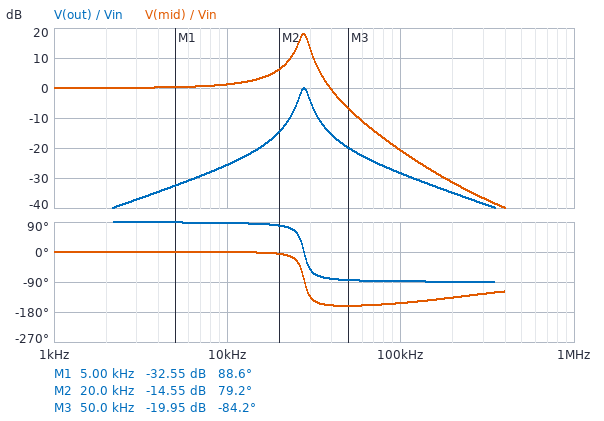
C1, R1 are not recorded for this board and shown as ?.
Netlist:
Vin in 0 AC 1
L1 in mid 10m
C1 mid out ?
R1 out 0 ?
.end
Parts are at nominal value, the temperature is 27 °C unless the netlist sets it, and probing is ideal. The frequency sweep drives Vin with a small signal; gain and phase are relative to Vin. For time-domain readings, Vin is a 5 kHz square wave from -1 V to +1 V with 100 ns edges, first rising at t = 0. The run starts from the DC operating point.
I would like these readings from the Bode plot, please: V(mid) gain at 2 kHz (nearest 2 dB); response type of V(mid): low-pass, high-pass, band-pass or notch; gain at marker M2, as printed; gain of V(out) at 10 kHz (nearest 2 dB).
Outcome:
0 dB
low-pass
-14.55 dB
-26 dB
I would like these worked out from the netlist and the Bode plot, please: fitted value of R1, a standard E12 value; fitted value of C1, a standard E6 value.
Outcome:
220 Ω
3.3 nF
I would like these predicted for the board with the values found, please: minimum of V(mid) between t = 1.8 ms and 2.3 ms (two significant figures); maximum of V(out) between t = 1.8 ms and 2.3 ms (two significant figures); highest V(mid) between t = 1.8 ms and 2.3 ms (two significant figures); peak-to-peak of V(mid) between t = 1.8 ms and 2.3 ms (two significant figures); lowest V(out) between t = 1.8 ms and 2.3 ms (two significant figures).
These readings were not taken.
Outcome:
-2.6 V
220 mV
2.6 V
5.1 V
-220 mV
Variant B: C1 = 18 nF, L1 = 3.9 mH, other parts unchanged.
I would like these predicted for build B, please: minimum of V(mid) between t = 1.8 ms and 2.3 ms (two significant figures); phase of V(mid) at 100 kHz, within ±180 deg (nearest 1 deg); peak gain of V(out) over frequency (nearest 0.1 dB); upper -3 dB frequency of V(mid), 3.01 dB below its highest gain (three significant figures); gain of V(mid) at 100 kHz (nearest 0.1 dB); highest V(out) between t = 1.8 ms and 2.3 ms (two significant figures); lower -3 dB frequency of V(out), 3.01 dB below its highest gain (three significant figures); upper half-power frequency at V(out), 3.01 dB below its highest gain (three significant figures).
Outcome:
-2.0 V
-107 deg
0 dB
22.4 kHz
-20.0 dB
670 mV
15.0 kHz
24.0 kHz
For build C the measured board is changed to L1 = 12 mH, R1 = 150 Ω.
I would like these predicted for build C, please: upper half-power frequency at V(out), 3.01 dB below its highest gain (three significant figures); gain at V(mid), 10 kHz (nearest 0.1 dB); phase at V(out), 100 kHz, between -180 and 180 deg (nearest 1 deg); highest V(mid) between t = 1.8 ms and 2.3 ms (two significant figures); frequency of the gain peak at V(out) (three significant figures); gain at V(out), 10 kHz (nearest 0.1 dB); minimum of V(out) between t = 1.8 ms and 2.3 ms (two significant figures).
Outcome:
26.3 kHz
1.5 dB
-89 deg
4.7 V
25.3 kHz
-28.7 dB
-310 mV
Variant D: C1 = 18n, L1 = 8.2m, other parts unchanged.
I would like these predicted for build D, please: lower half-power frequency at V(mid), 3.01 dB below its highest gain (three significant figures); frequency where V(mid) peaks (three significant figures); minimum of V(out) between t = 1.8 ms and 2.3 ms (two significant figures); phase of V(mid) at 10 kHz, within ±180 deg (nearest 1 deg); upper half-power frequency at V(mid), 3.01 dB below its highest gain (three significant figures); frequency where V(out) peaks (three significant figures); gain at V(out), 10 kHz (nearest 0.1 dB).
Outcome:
10.4 kHz
12.8 kHz
-510 mV
-17 deg
14.8 kHz
13.1 kHz
-5.8 dB
